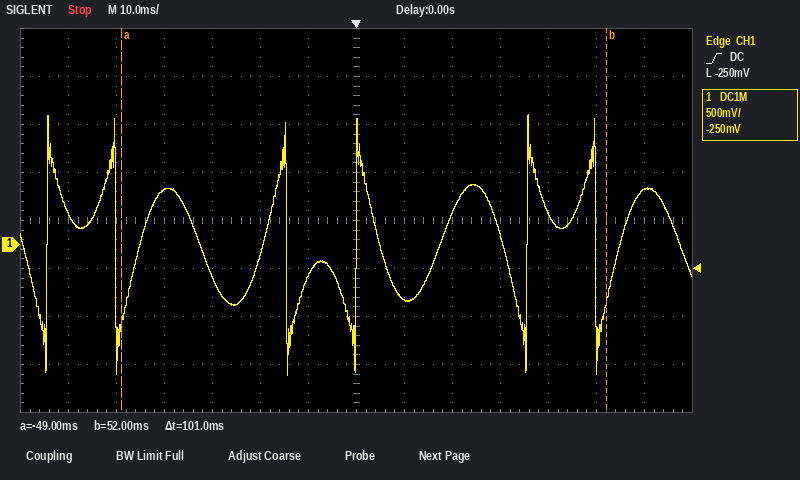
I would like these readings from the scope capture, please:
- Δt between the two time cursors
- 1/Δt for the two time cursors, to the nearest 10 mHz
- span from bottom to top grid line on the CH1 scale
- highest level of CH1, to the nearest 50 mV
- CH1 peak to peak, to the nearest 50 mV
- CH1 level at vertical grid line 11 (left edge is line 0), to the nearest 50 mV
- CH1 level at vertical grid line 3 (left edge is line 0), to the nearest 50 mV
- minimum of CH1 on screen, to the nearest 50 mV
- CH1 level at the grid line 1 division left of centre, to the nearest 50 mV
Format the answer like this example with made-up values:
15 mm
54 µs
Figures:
101 ms
9.90 Hz
4 V
1.35 V
2.70 V
350 mV
550 mV
-1.35 V
-350 mV
